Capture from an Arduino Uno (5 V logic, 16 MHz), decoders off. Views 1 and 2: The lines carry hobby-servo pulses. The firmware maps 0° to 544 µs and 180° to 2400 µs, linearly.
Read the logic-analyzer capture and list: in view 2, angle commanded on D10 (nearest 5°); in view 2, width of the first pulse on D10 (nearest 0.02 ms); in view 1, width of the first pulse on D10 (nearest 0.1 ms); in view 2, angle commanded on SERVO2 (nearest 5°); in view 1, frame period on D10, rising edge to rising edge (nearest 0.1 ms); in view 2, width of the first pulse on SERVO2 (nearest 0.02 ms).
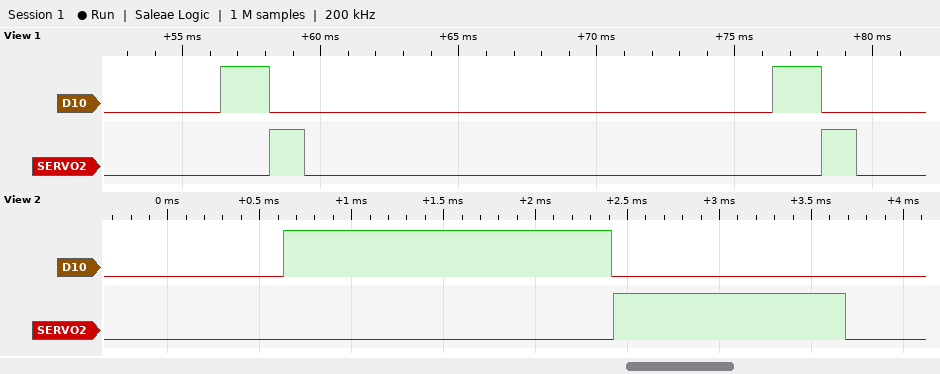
120°
1.78 ms
1.8 ms
70°
20.0 ms
1.26 ms
